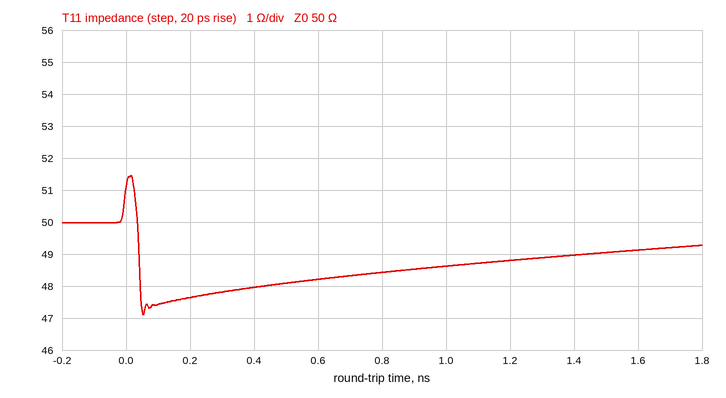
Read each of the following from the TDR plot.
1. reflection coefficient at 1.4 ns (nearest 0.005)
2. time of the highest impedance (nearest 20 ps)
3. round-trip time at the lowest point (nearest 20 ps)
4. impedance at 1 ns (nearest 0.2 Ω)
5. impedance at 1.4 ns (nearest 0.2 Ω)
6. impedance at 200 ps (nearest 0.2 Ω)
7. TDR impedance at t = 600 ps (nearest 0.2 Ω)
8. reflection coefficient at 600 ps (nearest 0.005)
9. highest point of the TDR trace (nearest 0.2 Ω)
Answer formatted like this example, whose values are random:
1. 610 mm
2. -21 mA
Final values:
1. -0.010
2. 20 ps
3. 60 ps
4. 48.6 Ω
5. 49.0 Ω
6. 47.6 Ω
7. 48.2 Ω
8. -0.020
9. 51.4 Ω
